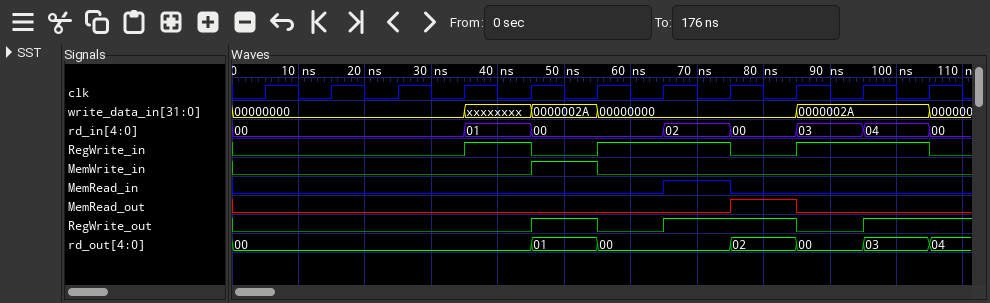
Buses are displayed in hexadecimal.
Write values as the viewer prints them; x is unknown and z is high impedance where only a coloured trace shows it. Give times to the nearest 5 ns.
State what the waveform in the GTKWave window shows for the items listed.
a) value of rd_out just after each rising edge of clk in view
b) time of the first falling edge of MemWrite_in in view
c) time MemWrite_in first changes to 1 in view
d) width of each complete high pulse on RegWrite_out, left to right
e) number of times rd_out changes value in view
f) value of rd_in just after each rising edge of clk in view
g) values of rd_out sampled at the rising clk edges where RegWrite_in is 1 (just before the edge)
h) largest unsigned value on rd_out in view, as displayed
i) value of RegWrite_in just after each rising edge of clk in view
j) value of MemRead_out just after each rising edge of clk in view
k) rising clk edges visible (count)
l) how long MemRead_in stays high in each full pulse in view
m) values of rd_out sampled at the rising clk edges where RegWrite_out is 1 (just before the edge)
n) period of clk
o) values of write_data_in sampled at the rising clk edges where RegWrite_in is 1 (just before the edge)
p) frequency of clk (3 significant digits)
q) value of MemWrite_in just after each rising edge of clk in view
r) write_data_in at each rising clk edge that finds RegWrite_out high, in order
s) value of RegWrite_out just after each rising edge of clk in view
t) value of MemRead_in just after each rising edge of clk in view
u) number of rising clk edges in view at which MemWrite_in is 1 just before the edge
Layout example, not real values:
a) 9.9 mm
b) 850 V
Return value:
a) 00, 00, 00, 00, 01, 00, 00, 02, 00, 03, 04
b) 55 ns
c) 45 ns
d) 10 ns, 20 ns
e) 6
f) 00, 00, 00, 01, 00, 00, 02, 00, 03, 04, 00
g) 00, 00, 00, 00, 03
h) 04
i) 0 0 0 1 0 1 1 0 1 1 0
j) 0 0 0 0 0 0 0 1 0 0 0
k) 11
l) 10 ns
m) 01, 00, 02, 03
n) 10 ns
o) xxxxxxxx, 00000000, 00000000, 0000002A, 0000002A
p) 100 MHz
q) 0 0 0 0 1 0 0 0 0 0 0
r) 0000002A, 00000000, 00000000, 0000002A
s) 0 0 0 0 1 0 1 1 0 1 1
t) 0 0 0 0 0 0 1 0 0 0 0
u) 1
